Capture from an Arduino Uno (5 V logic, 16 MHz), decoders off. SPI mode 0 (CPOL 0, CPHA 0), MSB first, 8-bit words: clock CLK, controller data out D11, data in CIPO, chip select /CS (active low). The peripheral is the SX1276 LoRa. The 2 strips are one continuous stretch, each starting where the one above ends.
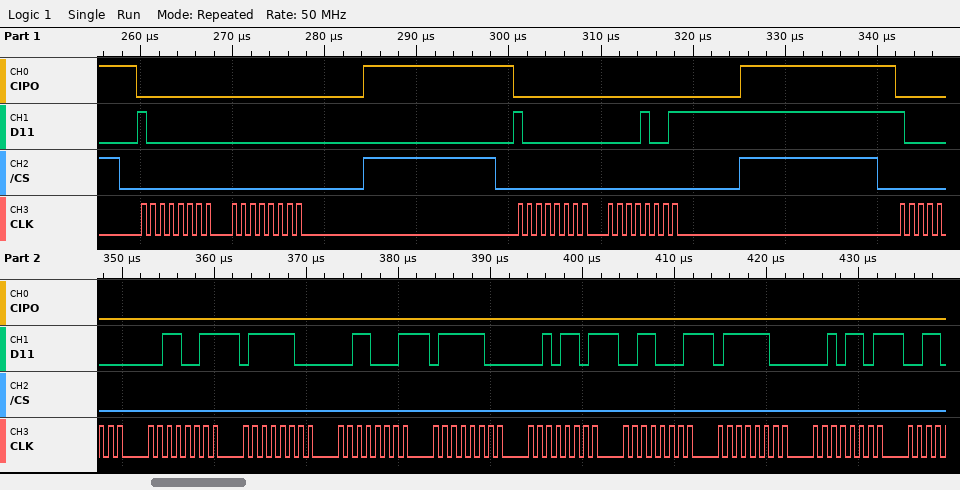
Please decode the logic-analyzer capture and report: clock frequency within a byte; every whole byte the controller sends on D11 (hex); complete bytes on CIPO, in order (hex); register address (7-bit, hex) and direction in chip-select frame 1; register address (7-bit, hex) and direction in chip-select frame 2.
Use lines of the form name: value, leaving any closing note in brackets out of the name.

clock frequency within a byte: 1 MHz
every whole byte the controller sends on D11: 80 00 80 09 80 33 7C 31 7C 2D 31 7C 2D
complete bytes on CIPO, in order: 00 00 00 00 00 00 00 00 00 00 00 00 00
register address (7-bit, hex) and direction in chip-select frame 1: 0x00 write
register address (7-bit, hex) and direction in chip-select frame 2: 0x00 write
